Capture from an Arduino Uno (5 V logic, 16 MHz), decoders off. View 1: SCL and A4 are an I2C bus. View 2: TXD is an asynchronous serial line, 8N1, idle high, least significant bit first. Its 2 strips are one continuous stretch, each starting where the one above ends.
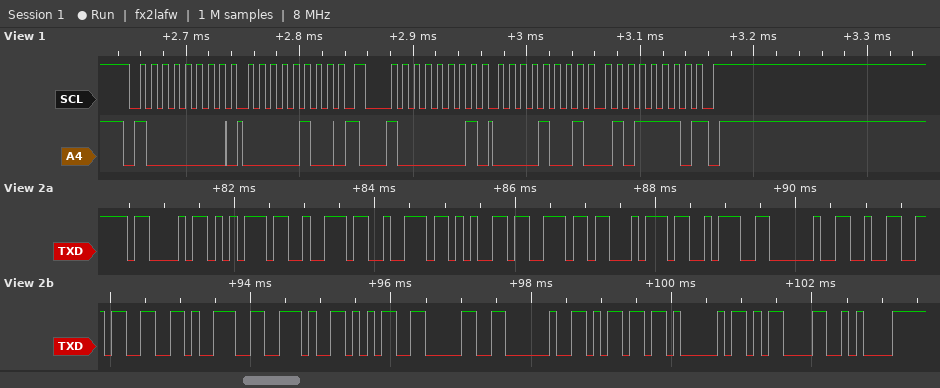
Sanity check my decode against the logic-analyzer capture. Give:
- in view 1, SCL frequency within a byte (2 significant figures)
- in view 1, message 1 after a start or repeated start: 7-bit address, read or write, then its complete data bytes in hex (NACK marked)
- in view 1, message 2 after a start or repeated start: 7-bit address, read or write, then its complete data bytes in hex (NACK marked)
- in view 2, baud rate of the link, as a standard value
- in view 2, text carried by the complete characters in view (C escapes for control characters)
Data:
100 kHz
0x40 write: 04
0x40 read: 09 5E NACK
9600 baud
"Current: 239.50 mA\r\n"
